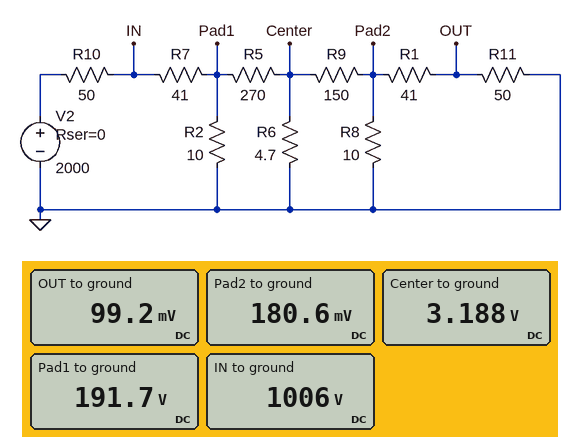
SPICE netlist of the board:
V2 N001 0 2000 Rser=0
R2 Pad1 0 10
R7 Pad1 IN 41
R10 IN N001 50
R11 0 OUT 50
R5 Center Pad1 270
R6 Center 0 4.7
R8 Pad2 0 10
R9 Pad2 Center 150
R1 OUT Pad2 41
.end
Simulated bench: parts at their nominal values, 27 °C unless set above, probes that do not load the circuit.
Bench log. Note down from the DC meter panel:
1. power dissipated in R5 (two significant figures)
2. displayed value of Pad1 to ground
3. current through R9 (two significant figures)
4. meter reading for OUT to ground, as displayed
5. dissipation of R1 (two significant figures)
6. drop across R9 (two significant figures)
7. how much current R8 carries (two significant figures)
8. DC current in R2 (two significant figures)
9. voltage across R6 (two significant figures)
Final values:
130 W
191.7 V
20 mA
99.2 mV
160 µW
3.0 V
18 mA
19 A
3.2 V
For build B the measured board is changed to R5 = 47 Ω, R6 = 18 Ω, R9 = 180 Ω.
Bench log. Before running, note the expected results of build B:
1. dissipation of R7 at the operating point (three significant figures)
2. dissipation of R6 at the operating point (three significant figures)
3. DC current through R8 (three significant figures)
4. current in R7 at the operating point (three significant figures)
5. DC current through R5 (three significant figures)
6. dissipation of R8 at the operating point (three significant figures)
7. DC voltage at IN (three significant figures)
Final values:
16.5 kW
112 W
214 mA
20.1 A
2.73 A
459 mW
996 V
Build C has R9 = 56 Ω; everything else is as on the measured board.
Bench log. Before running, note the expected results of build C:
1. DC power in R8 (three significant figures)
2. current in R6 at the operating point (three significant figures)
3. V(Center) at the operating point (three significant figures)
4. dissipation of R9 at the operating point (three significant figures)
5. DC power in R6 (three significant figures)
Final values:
18.0 mW
652 mA
3.06 V
124 mW
2.00 W
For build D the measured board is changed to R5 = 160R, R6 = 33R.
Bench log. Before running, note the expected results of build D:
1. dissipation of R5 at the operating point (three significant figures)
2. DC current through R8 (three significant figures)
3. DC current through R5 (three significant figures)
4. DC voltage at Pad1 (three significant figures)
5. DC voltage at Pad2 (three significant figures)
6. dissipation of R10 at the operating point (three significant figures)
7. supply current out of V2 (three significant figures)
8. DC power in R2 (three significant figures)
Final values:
163 W
156 mA
1.01 A
189 V
1.56 V
19.8 kW
19.9 A
3.57 kW
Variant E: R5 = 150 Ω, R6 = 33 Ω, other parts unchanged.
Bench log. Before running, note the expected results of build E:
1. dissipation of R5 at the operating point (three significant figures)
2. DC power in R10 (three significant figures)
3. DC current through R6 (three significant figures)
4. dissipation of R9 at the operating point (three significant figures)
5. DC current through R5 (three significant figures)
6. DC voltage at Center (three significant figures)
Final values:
169 W
19.8 kW
880 mA
5.00 W
1.06 A
29.0 V
